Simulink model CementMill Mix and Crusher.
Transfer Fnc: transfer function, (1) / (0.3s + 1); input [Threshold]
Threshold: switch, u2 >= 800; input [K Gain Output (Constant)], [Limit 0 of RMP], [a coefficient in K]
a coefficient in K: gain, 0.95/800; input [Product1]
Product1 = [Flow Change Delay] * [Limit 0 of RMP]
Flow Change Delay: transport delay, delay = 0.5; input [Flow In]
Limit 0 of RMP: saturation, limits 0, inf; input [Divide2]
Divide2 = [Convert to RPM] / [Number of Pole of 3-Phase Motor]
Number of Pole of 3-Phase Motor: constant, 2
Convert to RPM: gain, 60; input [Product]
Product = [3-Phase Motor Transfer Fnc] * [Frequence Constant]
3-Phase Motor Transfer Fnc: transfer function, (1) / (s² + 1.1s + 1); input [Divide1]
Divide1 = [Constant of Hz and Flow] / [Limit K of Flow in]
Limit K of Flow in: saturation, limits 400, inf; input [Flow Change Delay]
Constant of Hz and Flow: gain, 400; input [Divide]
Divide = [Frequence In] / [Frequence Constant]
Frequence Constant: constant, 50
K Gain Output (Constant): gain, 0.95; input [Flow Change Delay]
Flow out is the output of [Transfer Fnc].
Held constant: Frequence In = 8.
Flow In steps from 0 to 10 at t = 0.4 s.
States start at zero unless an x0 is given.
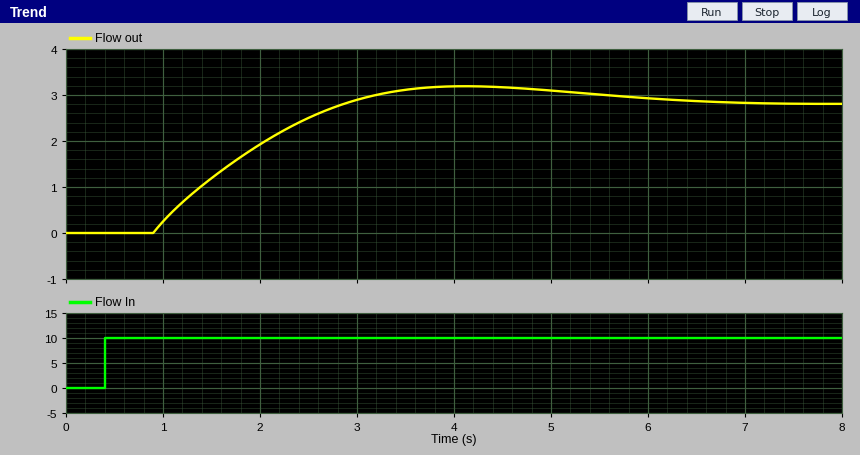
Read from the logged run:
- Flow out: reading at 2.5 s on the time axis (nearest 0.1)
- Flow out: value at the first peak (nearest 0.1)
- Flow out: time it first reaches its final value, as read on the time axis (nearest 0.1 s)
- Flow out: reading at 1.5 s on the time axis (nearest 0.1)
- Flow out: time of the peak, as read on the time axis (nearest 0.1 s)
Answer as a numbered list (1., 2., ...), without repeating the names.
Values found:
1. 2.5
2. 3.2
3. 2.9 s
4. 1.2
5. 4.1 s
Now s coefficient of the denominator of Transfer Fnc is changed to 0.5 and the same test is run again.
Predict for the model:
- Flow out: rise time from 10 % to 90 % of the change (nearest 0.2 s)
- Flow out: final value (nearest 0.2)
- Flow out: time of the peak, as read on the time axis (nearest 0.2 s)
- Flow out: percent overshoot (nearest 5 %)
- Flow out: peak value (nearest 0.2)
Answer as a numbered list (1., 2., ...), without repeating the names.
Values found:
1. 1.8 s
2. 2.8
3. 4.4 s
4. 10 %
5. 3.2
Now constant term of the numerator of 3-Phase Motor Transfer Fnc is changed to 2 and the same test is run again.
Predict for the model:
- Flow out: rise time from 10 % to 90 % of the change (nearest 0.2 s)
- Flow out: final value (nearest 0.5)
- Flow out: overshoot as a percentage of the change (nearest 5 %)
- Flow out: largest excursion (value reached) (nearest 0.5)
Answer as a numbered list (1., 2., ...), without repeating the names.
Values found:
1. 1.6 s
2. 5.5
3. 10 %
4. 6.5
